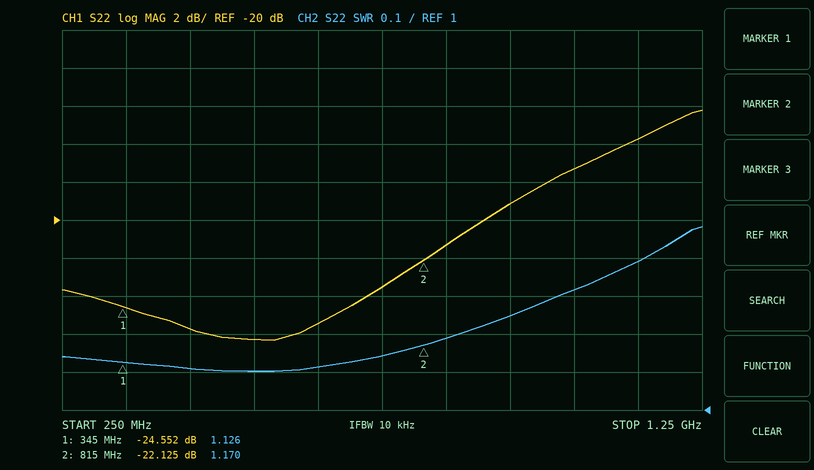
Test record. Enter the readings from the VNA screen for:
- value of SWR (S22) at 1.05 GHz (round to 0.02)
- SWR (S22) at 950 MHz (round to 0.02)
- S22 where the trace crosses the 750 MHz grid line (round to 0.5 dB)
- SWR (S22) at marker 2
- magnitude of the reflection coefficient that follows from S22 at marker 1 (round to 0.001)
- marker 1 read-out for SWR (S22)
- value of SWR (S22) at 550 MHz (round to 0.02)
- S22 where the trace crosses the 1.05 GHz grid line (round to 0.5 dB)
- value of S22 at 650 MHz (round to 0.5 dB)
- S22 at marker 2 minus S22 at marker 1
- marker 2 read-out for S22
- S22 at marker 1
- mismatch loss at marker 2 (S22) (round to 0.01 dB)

1.32
1.24
-23.5 dB
1.170
0.059
1.126
1.10
-17.5 dB
-25.5 dB
2.427 dB
-22.125 dB
-24.552 dB
0.03 dB
